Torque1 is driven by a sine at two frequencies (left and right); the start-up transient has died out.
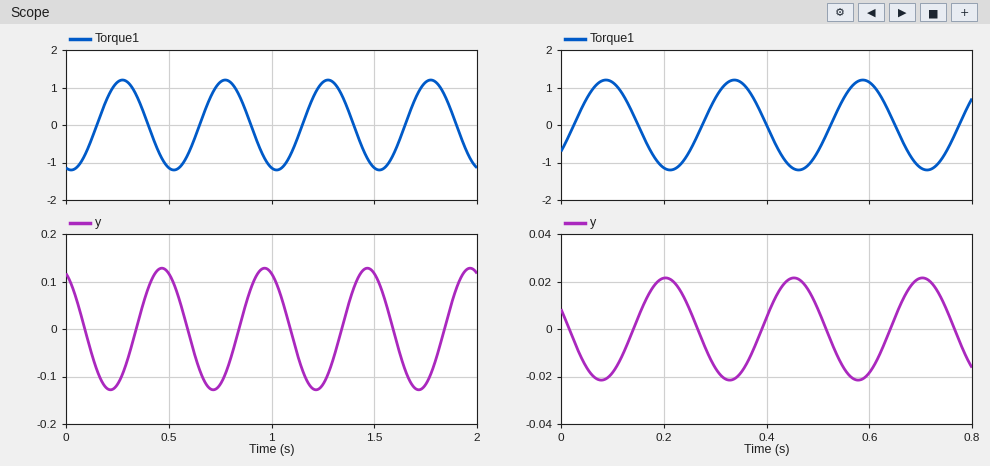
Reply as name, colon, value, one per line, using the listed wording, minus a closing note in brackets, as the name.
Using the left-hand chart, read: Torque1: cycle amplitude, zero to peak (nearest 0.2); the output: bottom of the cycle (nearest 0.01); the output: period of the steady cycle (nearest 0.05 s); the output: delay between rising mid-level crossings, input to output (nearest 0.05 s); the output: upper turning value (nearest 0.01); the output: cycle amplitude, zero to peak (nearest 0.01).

Torque1: cycle amplitude, zero to peak: 1.2
the output: bottom of the cycle: -0.13
the output: period of the steady cycle: 0.50 s
the output: delay between rising mid-level crossings, input to output: 0.20 s
the output: upper turning value: 0.13
the output: cycle amplitude, zero to peak: 0.13
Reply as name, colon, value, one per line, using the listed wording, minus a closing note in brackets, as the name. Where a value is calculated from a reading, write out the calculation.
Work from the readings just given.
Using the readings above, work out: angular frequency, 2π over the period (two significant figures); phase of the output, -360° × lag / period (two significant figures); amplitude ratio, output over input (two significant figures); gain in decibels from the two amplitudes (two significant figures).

angular frequency, 2π over the period: 2π / 0.5 = 13 rad/s
phase of the output, -360° × lag / period: -360 × 0.2 / 0.5 = -140°
amplitude ratio, output over input: 0.13 / 1.2 = 0.11
gain in decibels from the two amplitudes: 20 log10(0.13 / 1.2) = -19 dB
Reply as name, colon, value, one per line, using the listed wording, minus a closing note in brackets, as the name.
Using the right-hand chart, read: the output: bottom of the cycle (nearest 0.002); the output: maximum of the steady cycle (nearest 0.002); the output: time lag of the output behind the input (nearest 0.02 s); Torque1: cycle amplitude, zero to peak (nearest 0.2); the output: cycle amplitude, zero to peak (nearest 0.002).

the output: bottom of the cycle: -0.022
the output: maximum of the steady cycle: 0.022
the output: time lag of the output behind the input: 0.12 s
Torque1: cycle amplitude, zero to peak: 1.2
the output: cycle amplitude, zero to peak: 0.022
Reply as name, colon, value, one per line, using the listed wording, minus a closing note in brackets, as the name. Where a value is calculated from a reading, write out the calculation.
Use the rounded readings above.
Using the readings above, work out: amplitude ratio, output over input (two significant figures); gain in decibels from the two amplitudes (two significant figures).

amplitude ratio, output over input: 0.022 / 1.2 = 0.018
gain in decibels from the two amplitudes: 20 log10(0.022 / 1.2) = -35 dB
